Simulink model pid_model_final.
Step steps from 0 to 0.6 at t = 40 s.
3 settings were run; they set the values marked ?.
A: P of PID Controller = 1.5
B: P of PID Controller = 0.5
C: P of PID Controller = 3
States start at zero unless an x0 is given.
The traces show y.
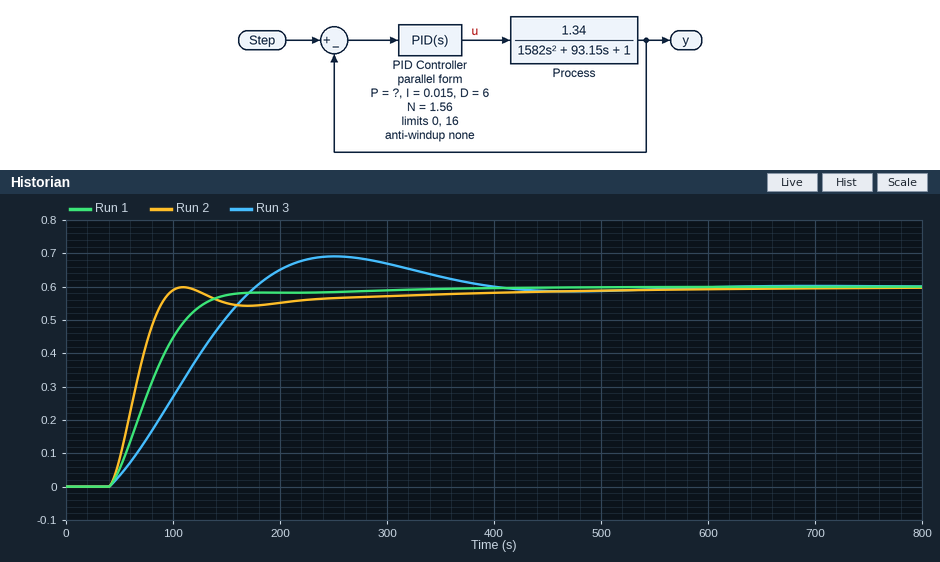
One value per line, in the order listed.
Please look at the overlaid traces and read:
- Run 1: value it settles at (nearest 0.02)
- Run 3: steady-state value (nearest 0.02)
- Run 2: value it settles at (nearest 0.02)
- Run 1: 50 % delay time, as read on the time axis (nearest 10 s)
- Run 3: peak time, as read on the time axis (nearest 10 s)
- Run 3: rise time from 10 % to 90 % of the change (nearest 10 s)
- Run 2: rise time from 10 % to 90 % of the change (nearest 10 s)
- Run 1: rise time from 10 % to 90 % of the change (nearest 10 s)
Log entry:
0.60
0.60
0.60
80 s
250 s
100 s
40 s
70 s
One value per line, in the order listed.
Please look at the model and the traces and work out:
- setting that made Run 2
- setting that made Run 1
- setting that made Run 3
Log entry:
C
A
B
